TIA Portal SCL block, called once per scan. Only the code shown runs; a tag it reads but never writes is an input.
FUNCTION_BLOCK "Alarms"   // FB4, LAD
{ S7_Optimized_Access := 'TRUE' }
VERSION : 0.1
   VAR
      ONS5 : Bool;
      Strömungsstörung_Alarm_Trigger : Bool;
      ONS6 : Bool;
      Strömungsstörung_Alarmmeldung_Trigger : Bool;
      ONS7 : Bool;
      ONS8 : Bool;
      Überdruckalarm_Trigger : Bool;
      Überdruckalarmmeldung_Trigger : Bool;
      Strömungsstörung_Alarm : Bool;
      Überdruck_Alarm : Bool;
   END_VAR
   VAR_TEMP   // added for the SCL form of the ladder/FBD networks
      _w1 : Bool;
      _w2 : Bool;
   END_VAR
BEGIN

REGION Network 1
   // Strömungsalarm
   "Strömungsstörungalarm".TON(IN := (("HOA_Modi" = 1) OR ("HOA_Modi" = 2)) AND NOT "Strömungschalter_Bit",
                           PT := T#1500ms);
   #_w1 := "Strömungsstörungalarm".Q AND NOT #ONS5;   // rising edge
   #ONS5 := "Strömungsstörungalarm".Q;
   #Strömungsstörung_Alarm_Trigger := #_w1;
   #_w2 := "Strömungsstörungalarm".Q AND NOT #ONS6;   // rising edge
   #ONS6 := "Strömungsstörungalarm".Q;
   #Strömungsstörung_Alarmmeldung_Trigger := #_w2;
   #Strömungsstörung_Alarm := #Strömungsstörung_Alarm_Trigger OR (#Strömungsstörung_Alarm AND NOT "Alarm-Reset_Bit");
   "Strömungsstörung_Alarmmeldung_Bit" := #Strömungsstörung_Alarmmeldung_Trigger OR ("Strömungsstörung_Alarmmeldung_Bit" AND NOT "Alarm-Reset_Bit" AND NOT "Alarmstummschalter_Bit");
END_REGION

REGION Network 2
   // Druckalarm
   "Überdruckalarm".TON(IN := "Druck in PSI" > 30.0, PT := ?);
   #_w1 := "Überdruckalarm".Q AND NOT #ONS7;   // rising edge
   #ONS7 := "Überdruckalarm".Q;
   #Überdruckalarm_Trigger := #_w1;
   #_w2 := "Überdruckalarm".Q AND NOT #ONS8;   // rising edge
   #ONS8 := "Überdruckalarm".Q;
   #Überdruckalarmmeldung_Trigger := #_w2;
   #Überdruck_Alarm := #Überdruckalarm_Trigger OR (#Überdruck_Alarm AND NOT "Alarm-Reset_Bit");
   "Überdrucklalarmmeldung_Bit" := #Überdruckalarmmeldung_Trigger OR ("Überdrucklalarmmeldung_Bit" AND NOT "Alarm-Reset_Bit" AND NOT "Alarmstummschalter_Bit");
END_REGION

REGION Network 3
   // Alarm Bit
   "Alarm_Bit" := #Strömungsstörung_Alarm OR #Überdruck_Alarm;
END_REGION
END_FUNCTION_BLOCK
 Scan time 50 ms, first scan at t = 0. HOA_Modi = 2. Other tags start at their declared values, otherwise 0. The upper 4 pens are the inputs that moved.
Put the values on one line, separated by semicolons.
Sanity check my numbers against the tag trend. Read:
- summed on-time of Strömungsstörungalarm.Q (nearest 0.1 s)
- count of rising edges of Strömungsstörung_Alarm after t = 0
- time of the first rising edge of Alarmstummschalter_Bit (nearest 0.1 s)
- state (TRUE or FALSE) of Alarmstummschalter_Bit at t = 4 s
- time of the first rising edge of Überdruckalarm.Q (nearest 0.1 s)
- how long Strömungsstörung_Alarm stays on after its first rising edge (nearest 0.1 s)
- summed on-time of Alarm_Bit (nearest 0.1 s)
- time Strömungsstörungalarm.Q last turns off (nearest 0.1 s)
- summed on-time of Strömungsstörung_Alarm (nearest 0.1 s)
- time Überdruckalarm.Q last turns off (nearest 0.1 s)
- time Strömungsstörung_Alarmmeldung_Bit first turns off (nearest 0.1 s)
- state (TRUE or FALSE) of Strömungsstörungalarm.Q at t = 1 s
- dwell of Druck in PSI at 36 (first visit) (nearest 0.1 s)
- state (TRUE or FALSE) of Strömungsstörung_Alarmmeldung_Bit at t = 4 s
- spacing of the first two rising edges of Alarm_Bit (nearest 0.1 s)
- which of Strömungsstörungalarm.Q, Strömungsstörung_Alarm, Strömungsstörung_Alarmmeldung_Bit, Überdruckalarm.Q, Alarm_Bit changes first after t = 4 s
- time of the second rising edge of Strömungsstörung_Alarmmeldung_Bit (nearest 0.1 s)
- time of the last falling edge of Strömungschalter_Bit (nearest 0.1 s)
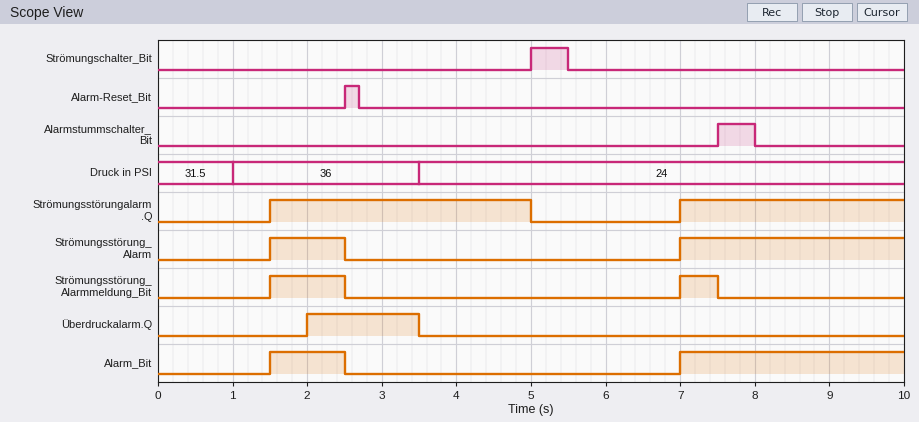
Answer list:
6.5 s; 2; 7.5 s; FALSE; 2.0 s; 1.0 s; 4.0 s; 5.0 s; 4.0 s; 3.5 s; 2.5 s; FALSE; 2.5 s; FALSE; 5.5 s; Strömungsstörungalarm.Q; 7.0 s; 5.5 s
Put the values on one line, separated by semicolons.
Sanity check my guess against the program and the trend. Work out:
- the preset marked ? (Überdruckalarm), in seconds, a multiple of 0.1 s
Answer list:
2.0 s
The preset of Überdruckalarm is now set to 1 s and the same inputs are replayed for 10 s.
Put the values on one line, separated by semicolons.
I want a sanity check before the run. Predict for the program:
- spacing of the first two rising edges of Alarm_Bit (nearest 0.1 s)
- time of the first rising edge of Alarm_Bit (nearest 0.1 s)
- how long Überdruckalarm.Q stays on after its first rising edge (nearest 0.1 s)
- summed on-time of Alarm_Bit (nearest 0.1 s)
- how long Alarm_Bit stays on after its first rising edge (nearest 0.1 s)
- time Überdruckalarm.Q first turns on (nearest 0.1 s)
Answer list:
6.0 s; 1.0 s; 2.5 s; 4.5 s; 1.5 s; 1.0 s
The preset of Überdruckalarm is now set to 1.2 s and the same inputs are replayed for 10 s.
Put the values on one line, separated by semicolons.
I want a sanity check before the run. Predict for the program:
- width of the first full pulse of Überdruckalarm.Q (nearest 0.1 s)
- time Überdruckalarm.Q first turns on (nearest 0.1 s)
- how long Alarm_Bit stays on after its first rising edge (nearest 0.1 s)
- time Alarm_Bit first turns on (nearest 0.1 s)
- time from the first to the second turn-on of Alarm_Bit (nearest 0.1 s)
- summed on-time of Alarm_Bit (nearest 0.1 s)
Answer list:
2.3 s; 1.2 s; 1.3 s; 1.2 s; 5.8 s; 4.3 s
